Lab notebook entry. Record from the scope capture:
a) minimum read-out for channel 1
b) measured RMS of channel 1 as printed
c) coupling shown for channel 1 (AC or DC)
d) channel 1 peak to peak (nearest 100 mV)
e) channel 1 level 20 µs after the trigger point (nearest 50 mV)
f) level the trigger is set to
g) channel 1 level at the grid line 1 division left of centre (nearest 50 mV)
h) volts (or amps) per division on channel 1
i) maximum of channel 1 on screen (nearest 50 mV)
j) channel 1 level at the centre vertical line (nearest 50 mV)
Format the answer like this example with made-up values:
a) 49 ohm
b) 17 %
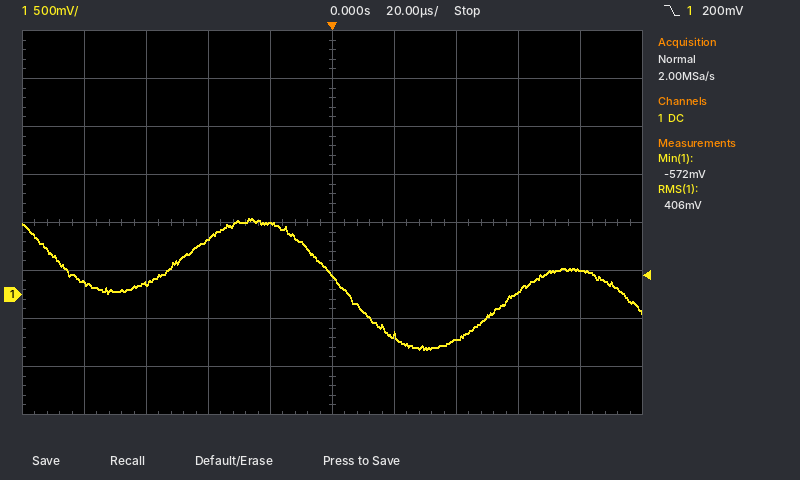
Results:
a) -572 mV
b) 406 mV
c) DC
d) 1.40 V
e) -450 mV
f) 200 mV
g) 750 mV
h) 500 mV
i) 800 mV
j) 200 mV
